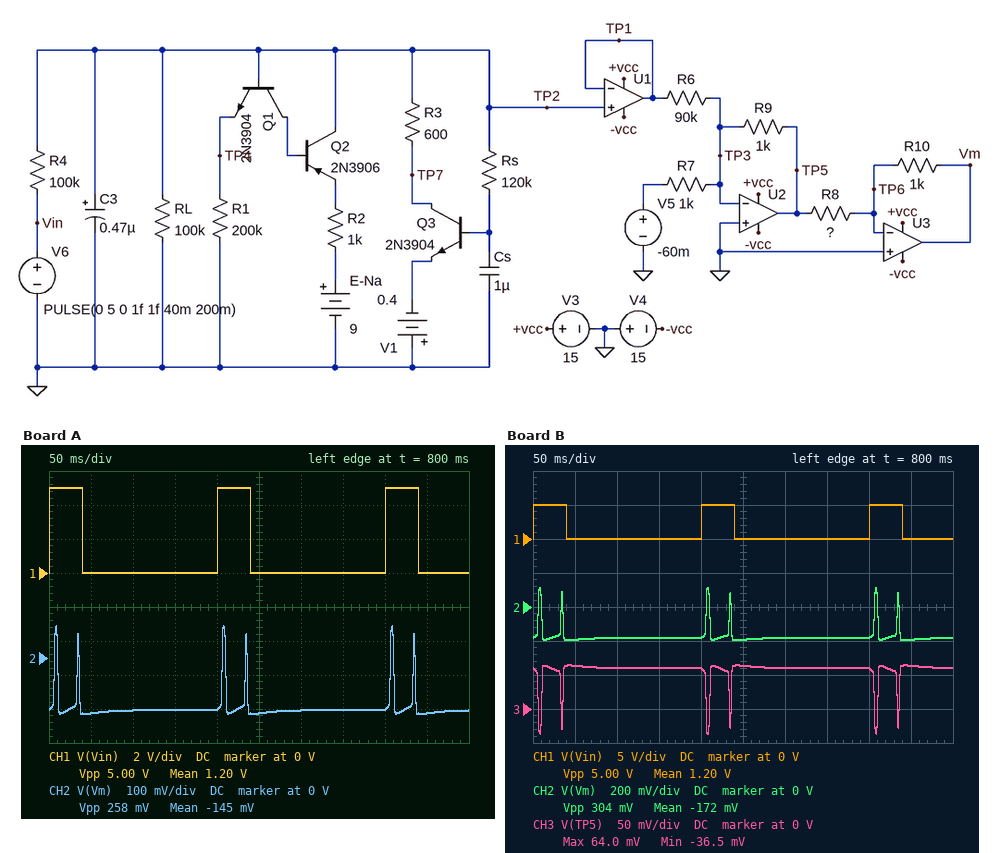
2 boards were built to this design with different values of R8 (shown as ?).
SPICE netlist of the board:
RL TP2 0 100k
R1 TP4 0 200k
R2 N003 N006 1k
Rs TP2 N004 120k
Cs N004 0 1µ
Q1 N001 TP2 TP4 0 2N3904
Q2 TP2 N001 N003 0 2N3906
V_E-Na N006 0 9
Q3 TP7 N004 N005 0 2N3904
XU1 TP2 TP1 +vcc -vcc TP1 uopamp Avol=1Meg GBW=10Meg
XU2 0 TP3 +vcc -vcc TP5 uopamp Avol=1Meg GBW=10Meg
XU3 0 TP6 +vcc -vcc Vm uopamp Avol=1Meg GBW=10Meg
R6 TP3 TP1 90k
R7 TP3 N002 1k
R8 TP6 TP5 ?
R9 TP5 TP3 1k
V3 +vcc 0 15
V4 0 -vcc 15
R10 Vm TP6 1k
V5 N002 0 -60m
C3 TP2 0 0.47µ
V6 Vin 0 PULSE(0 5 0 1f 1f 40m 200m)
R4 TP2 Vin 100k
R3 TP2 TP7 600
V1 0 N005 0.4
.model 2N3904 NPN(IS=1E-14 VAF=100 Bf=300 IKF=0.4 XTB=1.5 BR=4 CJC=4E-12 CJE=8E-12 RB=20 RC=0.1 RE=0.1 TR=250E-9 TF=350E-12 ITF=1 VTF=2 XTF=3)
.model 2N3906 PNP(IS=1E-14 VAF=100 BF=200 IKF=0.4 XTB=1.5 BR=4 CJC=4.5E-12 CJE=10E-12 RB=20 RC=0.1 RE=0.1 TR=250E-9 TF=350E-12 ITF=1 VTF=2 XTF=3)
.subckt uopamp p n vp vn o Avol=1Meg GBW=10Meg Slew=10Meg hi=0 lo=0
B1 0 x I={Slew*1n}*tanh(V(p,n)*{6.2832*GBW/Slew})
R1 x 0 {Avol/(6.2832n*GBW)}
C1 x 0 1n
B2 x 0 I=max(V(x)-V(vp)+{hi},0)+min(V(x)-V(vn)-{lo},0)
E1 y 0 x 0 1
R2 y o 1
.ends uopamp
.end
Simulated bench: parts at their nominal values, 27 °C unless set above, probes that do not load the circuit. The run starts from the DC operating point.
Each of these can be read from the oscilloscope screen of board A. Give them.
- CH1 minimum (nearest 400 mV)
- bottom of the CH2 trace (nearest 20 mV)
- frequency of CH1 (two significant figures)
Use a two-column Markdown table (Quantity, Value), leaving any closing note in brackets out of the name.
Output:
| Quantity | Value |
|---|---|
| CH1 minimum | 0 V |
| bottom of the CH2 trace | -160 mV |
| frequency of CH1 | 5.0 Hz |
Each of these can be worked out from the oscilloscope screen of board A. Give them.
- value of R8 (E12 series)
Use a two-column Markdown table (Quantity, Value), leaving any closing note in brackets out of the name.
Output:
| Quantity | Value |
|---|---|
| value of R8 | 390 Ω |
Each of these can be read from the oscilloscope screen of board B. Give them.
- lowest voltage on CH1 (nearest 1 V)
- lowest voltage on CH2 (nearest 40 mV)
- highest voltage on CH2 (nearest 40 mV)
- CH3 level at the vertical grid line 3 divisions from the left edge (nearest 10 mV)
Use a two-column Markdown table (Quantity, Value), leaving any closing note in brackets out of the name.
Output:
| Quantity | Value |
|---|---|
| lowest voltage on CH1 | 0 V |
| lowest voltage on CH2 | -200 mV |
| highest voltage on CH2 | 120 mV |
| CH3 level at the vertical grid line 3 divisions from the left edge | 60 mV |
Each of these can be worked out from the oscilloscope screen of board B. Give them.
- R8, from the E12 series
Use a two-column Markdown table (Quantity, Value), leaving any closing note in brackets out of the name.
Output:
| Quantity | Value |
|---|---|
| R8, from the E12 series | 330 Ω |
